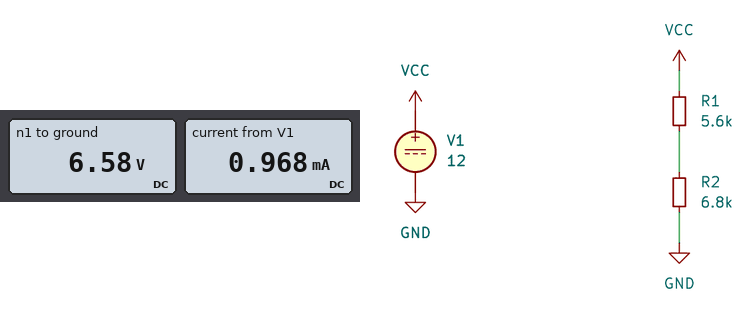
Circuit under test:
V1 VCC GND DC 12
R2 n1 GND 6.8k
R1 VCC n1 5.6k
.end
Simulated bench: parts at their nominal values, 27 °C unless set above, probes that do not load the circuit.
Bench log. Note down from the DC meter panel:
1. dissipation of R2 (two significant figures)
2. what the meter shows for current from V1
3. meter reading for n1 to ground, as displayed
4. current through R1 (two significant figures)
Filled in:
6.4 mW
0.968 mA
6.58 V
970 µA
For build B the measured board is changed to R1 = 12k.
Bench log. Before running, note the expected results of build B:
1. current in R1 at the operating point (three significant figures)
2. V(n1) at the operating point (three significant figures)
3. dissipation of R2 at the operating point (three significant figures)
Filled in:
638 µA
4.34 V
2.77 mW
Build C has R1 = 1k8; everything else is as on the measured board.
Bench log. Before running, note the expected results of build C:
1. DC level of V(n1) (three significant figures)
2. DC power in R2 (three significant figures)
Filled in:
9.49 V
13.2 mW
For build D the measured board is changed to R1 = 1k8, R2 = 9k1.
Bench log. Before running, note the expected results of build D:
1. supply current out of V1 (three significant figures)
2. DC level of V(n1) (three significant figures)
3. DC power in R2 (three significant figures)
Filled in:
1.10 mA
10.0 V
11.0 mW
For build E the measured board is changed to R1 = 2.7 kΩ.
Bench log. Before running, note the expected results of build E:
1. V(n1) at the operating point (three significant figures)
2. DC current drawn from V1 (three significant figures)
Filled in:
8.59 V
1.26 mA
